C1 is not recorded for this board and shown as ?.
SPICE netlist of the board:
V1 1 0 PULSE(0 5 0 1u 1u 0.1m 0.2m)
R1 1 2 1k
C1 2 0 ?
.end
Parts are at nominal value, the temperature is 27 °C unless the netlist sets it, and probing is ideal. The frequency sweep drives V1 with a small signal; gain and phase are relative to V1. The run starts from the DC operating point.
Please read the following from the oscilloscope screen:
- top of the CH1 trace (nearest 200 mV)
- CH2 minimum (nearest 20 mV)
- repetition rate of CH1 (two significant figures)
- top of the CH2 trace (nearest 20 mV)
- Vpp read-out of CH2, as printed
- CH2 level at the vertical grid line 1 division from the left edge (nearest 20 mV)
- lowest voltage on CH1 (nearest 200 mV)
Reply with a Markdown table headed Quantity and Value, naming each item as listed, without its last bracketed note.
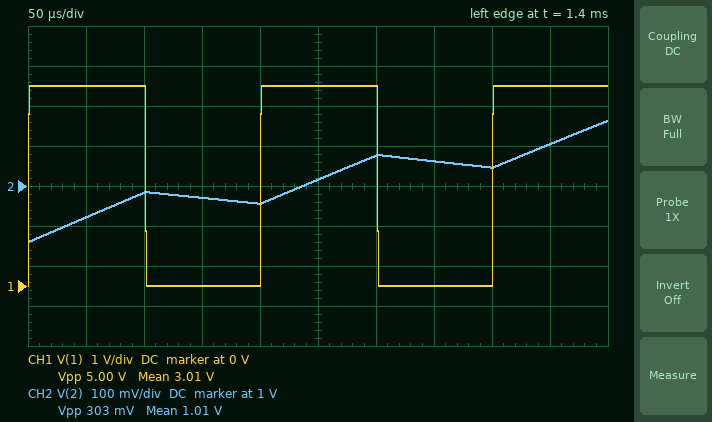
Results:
| Quantity | Value |
|---|---|
| top of the CH1 trace | 5.0 V |
| CH2 minimum | 860 mV |
| repetition rate of CH1 | 5.0 kHz |
| top of the CH2 trace | 1.16 V |
| Vpp read-out of CH2, as printed | 303 mV |
| CH2 level at the vertical grid line 1 division from the left edge | 920 mV |
| lowest voltage on CH1 | 0 V |
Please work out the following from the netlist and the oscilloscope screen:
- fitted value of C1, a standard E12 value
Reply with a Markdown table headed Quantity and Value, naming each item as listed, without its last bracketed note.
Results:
| Quantity | Value |
|---|---|
| fitted value of C1, a standard E12 value | 3.3 µF |
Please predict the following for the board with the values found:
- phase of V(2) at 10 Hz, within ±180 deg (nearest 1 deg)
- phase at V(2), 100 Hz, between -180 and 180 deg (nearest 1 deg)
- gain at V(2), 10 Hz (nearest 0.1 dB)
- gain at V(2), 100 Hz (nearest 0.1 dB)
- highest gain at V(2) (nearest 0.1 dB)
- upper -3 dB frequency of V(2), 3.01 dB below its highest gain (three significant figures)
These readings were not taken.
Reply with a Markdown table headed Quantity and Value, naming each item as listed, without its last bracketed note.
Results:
| Quantity | Value |
|---|---|
| phase of V(2) at 10 Hz, within ±180 deg | -12 deg |
| phase at V(2), 100 Hz, between -180 and 180 deg | -64 deg |
| gain at V(2), 10 Hz | -0.2 dB |
| gain at V(2), 100 Hz | -7.2 dB |
| highest gain at V(2) | 0 dB |
| upper -3 dB frequency of V(2), 3.01 dB below its highest gain | 48.2 Hz |
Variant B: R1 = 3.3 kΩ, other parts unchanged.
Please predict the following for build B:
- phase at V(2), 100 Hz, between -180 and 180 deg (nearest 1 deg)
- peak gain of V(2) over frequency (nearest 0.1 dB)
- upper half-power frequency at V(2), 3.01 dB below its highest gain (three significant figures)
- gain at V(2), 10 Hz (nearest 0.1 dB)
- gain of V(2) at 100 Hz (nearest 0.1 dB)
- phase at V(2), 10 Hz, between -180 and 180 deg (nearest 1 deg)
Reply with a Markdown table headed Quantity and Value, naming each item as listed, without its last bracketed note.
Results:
| Quantity | Value |
|---|---|
| phase at V(2), 100 Hz, between -180 and 180 deg | -82 deg |
| peak gain of V(2) over frequency | 0 dB |
| upper half-power frequency at V(2), 3.01 dB below its highest gain | 14.6 Hz |
| gain at V(2), 10 Hz | -1.7 dB |
| gain of V(2) at 100 Hz | -16.8 dB |
| phase at V(2), 10 Hz, between -180 and 180 deg | -34 deg |
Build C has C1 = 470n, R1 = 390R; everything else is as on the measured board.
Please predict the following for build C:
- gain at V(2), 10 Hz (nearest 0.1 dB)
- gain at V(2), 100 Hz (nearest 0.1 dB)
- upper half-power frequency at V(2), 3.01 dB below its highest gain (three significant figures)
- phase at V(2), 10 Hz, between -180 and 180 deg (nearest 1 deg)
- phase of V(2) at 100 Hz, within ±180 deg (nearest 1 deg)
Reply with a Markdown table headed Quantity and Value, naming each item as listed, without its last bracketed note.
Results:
| Quantity | Value |
|---|---|
| gain at V(2), 10 Hz | 0 dB |
| gain at V(2), 100 Hz | -0.1 dB |
| upper half-power frequency at V(2), 3.01 dB below its highest gain | 868 Hz |
| phase at V(2), 10 Hz, between -180 and 180 deg | -1 deg |
| phase of V(2) at 100 Hz, within ±180 deg | -7 deg |
